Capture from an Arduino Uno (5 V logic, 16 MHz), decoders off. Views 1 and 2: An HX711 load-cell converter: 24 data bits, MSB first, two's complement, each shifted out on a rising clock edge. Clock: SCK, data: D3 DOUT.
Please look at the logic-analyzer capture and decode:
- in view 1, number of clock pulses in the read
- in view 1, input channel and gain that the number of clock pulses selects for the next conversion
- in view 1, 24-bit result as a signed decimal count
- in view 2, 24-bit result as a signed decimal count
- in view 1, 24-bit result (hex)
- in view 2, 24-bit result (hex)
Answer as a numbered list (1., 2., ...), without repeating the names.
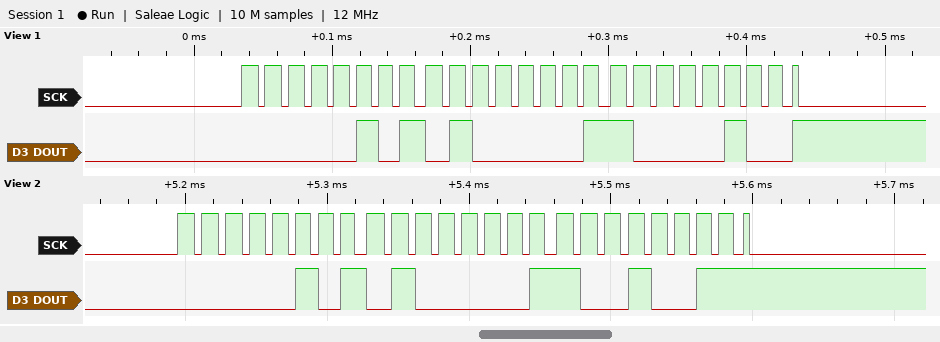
1. 25
2. channel A, gain 128
3. 344452
4. 344467
5. 0x054184
6. 0x054193
